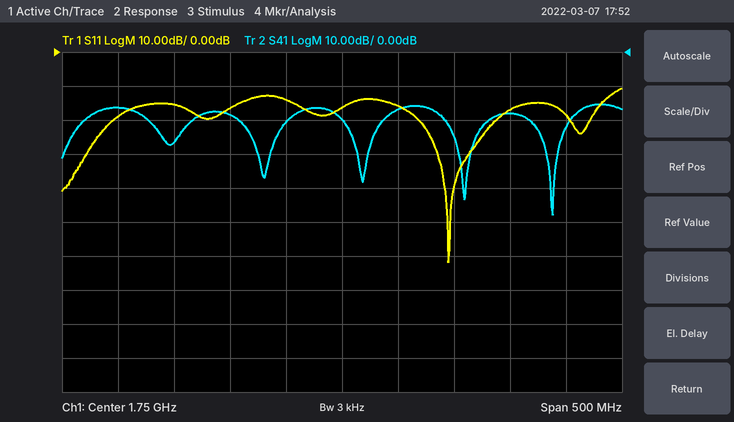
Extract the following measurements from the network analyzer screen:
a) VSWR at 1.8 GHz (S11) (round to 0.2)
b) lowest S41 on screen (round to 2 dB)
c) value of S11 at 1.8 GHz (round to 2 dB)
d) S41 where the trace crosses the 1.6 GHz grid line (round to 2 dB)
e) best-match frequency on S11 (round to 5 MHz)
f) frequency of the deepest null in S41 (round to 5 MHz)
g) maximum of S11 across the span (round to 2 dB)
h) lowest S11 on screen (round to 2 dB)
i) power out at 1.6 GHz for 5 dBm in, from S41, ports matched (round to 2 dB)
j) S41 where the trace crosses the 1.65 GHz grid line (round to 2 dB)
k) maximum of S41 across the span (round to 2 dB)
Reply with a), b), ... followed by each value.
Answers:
a) 1.4
b) -48 dB
c) -16 dB
d) -26 dB
e) 1.845 GHz
f) 1.940 GHz
g) -10 dB
h) -62 dB
i) -22 dBm
j) -18 dB
k) -16 dB
